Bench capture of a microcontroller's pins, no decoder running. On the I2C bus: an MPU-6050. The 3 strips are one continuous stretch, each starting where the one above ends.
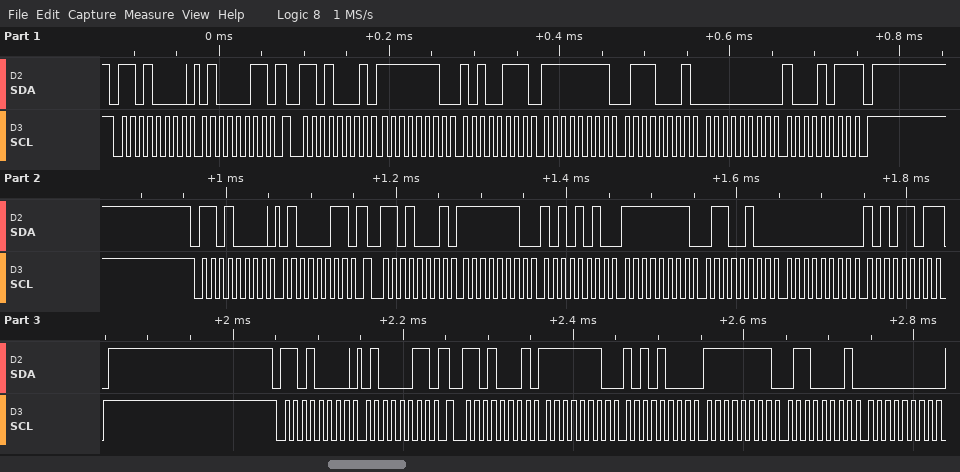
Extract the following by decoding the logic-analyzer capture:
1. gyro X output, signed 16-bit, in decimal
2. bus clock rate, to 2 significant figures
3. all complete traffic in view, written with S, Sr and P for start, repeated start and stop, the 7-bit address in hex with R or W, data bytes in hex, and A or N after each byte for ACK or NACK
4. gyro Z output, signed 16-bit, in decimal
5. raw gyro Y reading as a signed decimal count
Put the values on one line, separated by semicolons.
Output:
-345; 100 kHz; S 68W A 43 A Sr 68R A FE A A7 A FF A 71 A 00 A 8B N P S 68W A 43 A Sr 68R A FE A AA A FF A 64 A 00 A AD N P S 68W A 43 A Sr 68R A FE A A8 A FF A 61 A 00 A; 139; -143
